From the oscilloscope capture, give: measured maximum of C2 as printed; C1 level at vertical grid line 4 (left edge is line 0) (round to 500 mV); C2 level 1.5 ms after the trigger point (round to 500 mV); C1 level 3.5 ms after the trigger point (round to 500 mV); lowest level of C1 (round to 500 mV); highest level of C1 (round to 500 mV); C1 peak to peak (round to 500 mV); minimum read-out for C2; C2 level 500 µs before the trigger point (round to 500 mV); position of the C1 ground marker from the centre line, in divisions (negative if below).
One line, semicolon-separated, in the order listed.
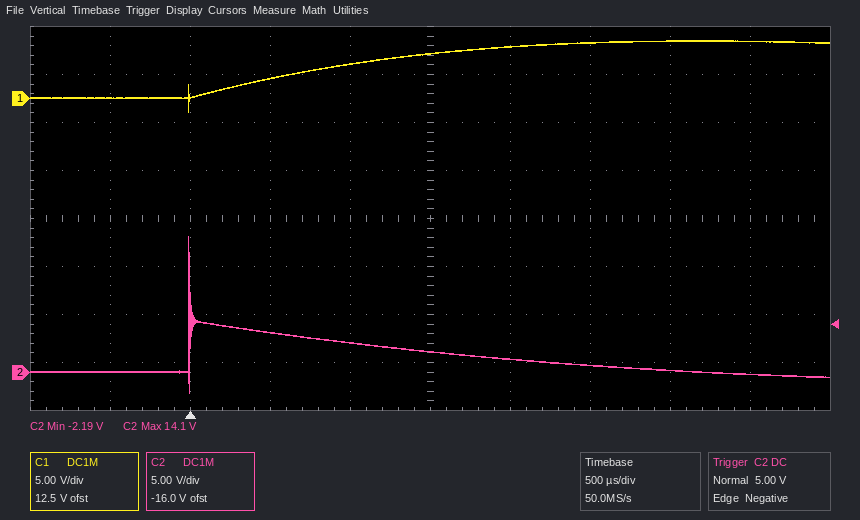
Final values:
14.1 V; 3.5 V; 2.0 V; 6.0 V; -1.5 V; 6.0 V; 7.5 V; -2.19 V; 0.0 V; +2.5 div
